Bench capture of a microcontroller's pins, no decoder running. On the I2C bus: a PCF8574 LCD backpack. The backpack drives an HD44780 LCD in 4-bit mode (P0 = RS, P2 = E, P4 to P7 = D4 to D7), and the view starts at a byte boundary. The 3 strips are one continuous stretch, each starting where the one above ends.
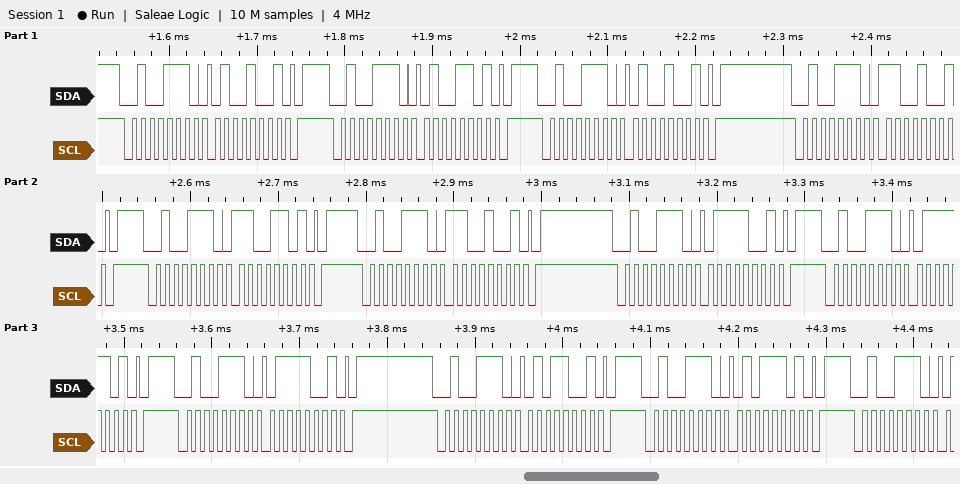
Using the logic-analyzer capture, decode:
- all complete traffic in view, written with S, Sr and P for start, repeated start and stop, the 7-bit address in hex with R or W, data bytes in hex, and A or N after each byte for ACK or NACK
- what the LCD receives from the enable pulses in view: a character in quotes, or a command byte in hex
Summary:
S 27W A 49 A P S 27W A 4D A P S 27W A 49 A P S 27W A C9 A P S 27W A CD A P S 27W A C9 A P S 27W A 79 A P S 27W A 7D A P S 27W A 79 A P S 27W A 59 A P S 27W A 5D A P S 27W A
'L'
